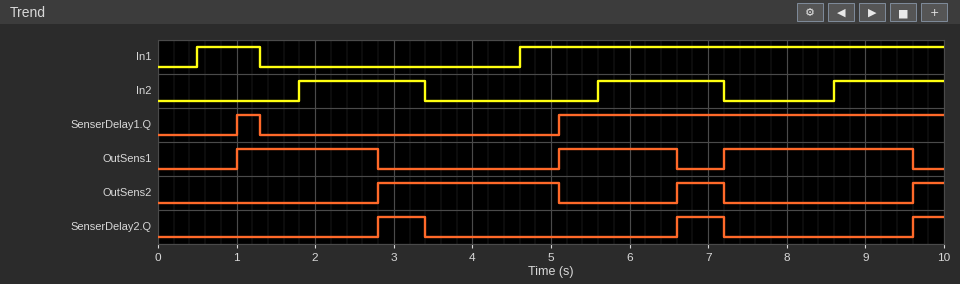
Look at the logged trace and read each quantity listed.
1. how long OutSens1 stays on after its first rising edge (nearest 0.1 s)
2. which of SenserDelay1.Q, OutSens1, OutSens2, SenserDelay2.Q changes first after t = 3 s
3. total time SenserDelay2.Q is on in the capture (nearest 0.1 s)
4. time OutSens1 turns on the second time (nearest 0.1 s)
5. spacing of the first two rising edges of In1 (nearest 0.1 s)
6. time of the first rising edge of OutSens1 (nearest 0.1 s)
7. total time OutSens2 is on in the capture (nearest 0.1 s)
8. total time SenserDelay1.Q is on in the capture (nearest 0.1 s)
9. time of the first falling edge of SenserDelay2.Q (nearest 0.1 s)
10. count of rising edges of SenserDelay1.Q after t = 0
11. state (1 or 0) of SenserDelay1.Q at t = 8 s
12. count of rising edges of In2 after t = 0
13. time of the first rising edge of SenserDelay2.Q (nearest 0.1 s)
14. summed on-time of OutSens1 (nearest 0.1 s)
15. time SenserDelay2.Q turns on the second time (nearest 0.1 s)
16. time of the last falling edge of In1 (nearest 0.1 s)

1.8 s
SenserDelay2.Q
1.6 s
5.1 s
4.1 s
1.0 s
3.3 s
5.2 s
3.4 s
2
1
3
2.8 s
5.7 s
6.6 s
1.3 s
